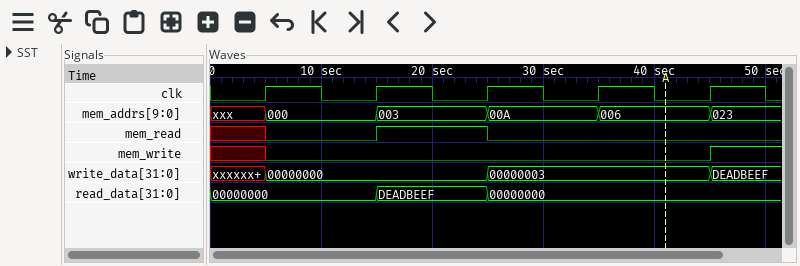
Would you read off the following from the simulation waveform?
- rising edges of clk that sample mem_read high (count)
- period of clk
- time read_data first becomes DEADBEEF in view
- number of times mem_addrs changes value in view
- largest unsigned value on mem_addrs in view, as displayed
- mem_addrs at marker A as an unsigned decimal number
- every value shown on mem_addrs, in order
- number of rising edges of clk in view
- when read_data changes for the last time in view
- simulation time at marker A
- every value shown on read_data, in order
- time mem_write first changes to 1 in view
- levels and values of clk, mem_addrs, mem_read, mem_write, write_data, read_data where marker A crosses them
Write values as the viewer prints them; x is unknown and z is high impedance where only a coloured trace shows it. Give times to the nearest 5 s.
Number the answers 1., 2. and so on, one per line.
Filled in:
1. 1
2. 10 s
3. 15 s
4. 5
5. 023
6. 6
7. xxx, 000, 003, 00A, 006, 023
8. 5
9. 25 s
10. 40 s
11. 00000000, DEADBEEF, 00000000
12. 45 s
13. clk=0, mem_addrs=006, mem_read=0, mem_write=0, write_data=00000003, read_data=00000000
